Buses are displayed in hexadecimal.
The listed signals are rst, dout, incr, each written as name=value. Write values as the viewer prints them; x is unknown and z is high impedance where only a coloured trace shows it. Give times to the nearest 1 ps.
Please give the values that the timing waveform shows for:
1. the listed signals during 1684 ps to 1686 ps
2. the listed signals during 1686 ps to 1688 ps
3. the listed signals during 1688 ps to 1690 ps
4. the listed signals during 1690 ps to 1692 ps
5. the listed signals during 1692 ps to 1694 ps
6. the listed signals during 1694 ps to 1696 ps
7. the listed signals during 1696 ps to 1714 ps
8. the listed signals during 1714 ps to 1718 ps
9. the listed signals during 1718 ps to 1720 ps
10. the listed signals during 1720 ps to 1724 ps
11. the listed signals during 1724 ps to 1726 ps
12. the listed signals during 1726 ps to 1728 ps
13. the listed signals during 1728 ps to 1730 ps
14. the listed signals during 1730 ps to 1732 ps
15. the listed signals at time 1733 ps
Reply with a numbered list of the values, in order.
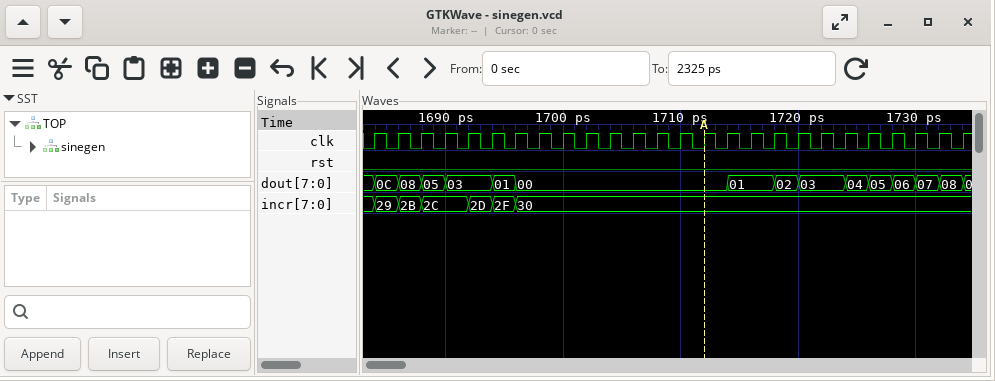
1. rst=0, dout=0C, incr=29
2. rst=0, dout=08, incr=2B
3. rst=0, dout=05, incr=2C
4. rst=0, dout=03, incr=2C
5. rst=0, dout=03, incr=2D
6. rst=0, dout=01, incr=2F
7. rst=0, dout=00, incr=30
8. rst=0, dout=01, incr=30
9. rst=0, dout=02, incr=30
10. rst=0, dout=03, incr=30
11. rst=0, dout=04, incr=30
12. rst=0, dout=05, incr=30
13. rst=0, dout=06, incr=30
14. rst=0, dout=07, incr=30
15. rst=0, dout=08, incr=30
